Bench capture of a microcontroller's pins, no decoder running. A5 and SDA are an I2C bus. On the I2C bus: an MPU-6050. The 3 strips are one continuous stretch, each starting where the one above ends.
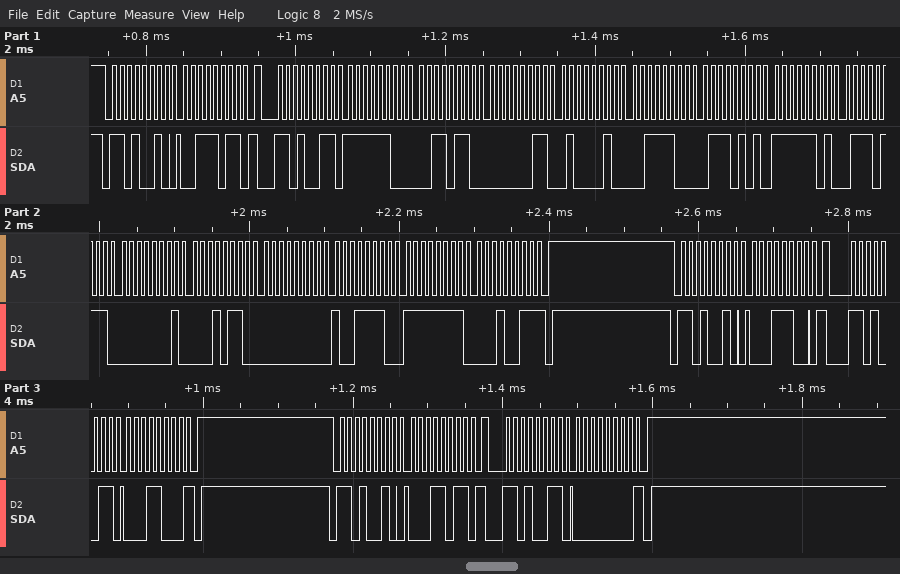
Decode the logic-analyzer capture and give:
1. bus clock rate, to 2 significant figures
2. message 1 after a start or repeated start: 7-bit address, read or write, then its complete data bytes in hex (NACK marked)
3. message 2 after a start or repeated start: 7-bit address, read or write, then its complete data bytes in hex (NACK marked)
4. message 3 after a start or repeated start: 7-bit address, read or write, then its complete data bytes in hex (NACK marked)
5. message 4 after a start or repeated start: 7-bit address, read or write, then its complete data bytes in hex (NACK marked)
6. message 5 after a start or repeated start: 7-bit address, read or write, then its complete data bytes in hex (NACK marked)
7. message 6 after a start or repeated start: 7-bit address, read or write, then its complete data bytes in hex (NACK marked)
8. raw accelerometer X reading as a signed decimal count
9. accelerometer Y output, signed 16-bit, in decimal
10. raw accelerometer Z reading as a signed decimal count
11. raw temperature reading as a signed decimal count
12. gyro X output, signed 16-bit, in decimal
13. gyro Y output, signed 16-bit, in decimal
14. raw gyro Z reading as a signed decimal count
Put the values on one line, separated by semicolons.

100 kHz; 0x69 write: 3B; 0x69 read: FC 36 03 42 3C 75 FD 77 01 16 00 9E FF 13 NACK; 0x69 write: 1C; 0x69 read: 18 NACK; 0x69 write: 1B; 0x69 read: 00 NACK; -970; 834; 15477; -649; 278; 158; -237
